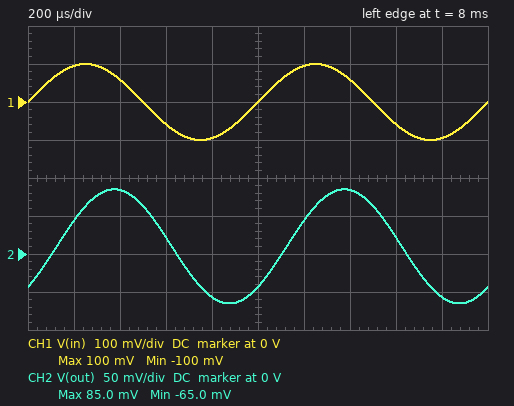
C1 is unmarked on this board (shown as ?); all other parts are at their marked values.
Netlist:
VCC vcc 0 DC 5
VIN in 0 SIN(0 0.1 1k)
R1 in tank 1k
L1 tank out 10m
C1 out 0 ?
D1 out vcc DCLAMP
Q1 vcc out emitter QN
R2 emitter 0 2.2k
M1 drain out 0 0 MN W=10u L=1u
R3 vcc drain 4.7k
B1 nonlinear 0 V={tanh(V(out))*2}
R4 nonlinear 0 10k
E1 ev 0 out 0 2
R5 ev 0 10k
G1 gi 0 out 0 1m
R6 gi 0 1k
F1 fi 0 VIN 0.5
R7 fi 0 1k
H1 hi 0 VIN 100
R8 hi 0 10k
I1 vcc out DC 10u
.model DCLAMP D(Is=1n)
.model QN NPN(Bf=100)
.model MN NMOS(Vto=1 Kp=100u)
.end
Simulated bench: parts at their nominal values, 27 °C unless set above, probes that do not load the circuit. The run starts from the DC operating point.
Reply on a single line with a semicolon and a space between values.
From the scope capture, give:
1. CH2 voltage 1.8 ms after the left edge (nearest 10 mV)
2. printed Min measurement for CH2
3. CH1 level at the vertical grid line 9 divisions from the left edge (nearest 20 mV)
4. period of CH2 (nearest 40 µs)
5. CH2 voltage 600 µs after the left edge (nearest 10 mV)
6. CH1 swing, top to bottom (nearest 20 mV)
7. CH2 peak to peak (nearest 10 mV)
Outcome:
-60 mV; -65.0 mV; -100 mV; 1.00 ms; 20 mV; 200 mV; 150 mV
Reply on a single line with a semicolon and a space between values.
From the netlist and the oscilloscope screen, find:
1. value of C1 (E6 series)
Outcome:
150 nF
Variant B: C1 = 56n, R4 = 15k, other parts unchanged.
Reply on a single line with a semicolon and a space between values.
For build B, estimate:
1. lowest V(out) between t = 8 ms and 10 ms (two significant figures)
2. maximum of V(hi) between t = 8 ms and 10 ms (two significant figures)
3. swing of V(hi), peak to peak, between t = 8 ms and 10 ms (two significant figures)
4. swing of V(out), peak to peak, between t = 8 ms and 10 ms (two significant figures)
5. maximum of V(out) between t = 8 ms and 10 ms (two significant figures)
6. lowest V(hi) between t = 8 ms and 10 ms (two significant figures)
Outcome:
-86 mV; 4.4 mV; 6.8 mV; 190 mV; 110 mV; -2.4 mV
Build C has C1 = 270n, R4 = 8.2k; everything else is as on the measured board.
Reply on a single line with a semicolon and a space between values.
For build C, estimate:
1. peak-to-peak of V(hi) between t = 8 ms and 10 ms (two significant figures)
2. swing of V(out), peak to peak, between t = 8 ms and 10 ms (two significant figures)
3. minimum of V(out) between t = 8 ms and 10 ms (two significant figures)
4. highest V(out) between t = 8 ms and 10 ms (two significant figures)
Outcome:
18 mV; 100 mV; -42 mV; 62 mV
